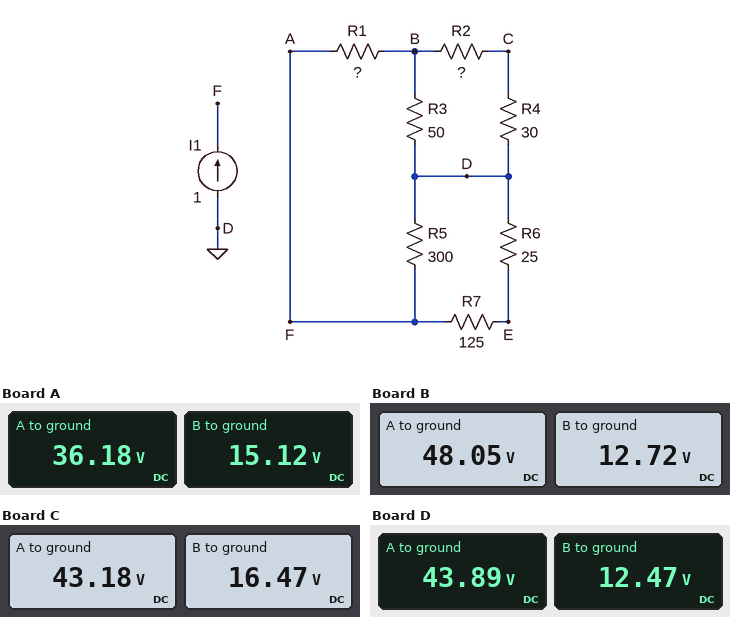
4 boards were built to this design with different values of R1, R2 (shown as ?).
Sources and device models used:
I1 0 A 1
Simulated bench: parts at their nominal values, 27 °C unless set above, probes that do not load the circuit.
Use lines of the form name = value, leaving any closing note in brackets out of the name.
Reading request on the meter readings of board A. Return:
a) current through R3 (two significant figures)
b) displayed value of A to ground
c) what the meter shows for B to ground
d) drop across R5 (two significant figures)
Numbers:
current through R3 = 300 mA
displayed value of A to ground = 36.18 V
what the meter shows for B to ground = 15.12 V
drop across R5 = 36 V
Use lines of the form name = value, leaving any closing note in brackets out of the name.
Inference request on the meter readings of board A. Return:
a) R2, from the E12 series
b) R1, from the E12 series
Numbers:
R2, from the E12 series = 15 Ω
R1, from the E12 series = 33 Ω
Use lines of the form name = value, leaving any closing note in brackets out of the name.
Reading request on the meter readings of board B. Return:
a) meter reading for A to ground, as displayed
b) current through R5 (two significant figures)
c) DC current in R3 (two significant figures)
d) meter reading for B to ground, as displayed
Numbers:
meter reading for A to ground, as displayed = 48.05 V
current through R5 = 160 mA
DC current in R3 = 250 mA
meter reading for B to ground, as displayed = 12.72 V
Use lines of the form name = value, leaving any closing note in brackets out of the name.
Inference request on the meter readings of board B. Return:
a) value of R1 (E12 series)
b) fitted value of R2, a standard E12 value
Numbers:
value of R1 = 68 Ω
fitted value of R2, a standard E12 value = 18 Ω
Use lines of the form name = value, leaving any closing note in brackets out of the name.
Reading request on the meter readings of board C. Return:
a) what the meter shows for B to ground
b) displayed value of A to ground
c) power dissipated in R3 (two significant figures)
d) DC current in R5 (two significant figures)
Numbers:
what the meter shows for B to ground = 16.47 V
displayed value of A to ground = 43.18 V
power dissipated in R3 = 5.4 W
DC current in R5 = 140 mA
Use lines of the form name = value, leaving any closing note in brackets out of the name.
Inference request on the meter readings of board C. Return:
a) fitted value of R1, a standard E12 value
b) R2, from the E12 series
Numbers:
fitted value of R1, a standard E12 value = 47 Ω
R2, from the E12 series = 39 Ω
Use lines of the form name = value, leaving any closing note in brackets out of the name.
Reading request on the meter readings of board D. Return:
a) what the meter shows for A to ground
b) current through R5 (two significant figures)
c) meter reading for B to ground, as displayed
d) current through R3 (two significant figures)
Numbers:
what the meter shows for A to ground = 43.89 V
current through R5 = 150 mA
meter reading for B to ground, as displayed = 12.47 V
current through R3 = 250 mA
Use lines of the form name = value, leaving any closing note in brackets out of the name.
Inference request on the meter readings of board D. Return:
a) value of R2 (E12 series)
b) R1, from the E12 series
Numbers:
value of R2 = 10 Ω
R1, from the E12 series = 56 Ω
